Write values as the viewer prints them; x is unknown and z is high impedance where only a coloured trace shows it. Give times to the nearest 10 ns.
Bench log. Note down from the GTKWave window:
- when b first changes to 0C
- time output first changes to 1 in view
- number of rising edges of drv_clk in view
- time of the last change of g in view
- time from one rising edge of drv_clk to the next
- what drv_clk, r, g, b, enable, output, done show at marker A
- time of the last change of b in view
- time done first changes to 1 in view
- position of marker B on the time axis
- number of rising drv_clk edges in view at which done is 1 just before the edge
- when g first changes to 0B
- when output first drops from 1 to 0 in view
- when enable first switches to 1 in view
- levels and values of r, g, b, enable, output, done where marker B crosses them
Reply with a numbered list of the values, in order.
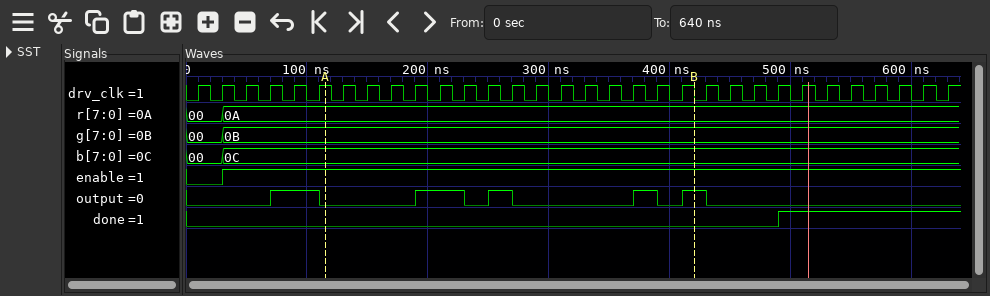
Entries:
1. 30 ns
2. 70 ns
3. 32
4. 30 ns
5. 20 ns
6. drv_clk=1, r=0A, g=0B, b=0C, enable=1, output=0, done=0
7. 30 ns
8. 490 ns
9. 420 ns
10. 7
11. 30 ns
12. 110 ns
13. 30 ns
14. r=0A, g=0B, b=0C, enable=1, output=1, done=0
